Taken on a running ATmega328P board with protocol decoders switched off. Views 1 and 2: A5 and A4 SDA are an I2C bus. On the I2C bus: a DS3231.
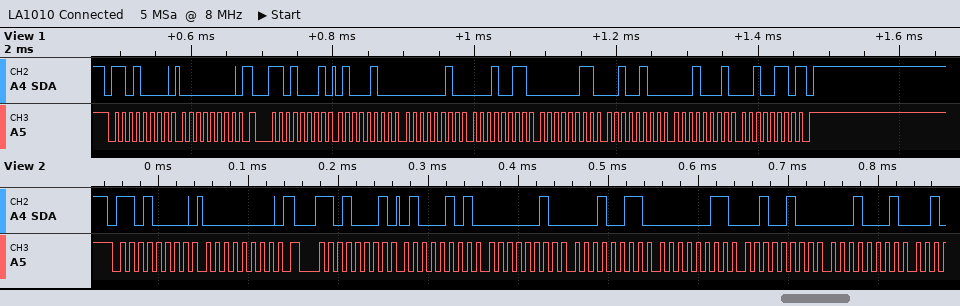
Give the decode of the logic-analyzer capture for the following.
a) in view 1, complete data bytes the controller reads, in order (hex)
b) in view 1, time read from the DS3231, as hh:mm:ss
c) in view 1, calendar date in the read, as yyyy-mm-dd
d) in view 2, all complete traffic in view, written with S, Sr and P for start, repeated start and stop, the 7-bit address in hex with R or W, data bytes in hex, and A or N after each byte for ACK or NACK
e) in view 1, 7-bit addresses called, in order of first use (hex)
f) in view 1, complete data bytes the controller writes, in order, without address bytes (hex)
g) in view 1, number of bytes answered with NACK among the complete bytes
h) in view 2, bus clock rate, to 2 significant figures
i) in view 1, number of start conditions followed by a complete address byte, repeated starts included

44 02 13 03 24 11 26
13:02:44
2026-11-24
S 68W A 00 A Sr 68R A 45 A 02 A 13 A 03 A 24 A 11 A
0x68
00
1
100 kHz
2
